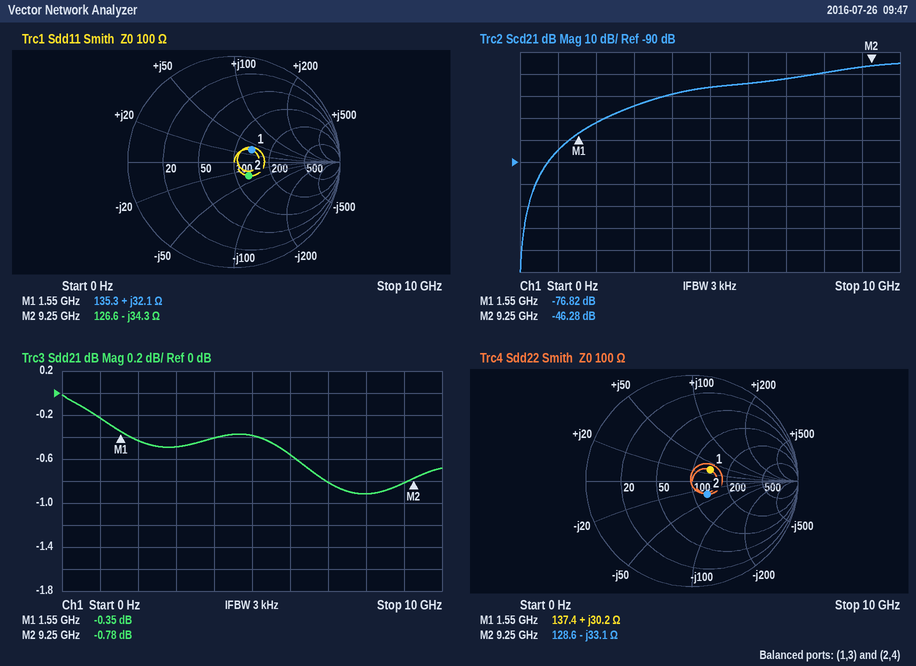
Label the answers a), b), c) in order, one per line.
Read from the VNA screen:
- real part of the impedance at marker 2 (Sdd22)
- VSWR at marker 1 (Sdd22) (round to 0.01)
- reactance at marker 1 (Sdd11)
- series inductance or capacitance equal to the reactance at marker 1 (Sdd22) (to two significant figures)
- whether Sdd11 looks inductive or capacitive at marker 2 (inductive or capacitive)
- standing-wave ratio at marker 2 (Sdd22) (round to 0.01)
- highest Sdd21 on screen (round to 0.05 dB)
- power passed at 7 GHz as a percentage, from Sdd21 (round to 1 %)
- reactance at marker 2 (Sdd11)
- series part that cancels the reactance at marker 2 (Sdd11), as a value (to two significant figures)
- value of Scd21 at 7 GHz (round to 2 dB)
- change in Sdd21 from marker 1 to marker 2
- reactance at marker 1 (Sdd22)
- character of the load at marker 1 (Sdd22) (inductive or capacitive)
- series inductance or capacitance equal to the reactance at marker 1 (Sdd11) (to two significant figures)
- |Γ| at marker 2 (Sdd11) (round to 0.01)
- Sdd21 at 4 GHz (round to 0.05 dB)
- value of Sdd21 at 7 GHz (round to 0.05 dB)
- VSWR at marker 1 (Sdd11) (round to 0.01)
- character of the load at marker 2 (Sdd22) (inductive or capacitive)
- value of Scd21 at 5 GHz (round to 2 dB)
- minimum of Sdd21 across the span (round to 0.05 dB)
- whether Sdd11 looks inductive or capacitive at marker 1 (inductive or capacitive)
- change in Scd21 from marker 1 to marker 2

a) 128.6 Ω
b) 1.50
c) +32.1 Ω
d) 3.1 nH
e) capacitive
f) 1.47
g) 0.00 dB
h) 83 %
i) -34.3 Ω
j) 590 pH
k) -52 dB
l) -0.43 dB
m) +30.2 Ω
n) inductive
o) 3.3 nH
p) 0.19
q) -0.40 dB
r) -0.80 dB
s) 1.50
t) capacitive
u) -56 dB
v) -0.90 dB
w) inductive
x) 30.54 dB
